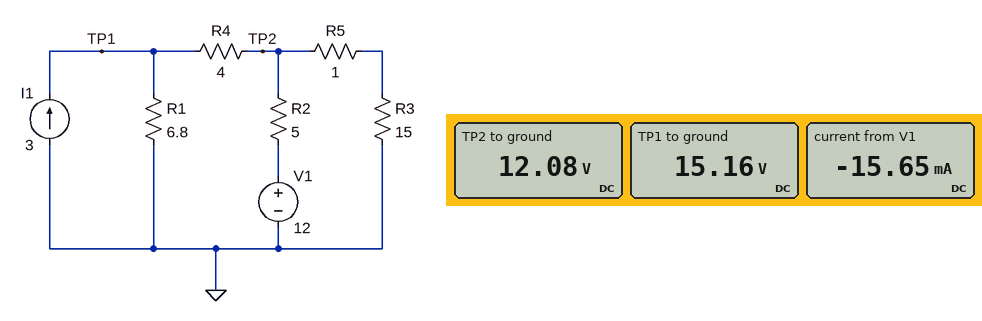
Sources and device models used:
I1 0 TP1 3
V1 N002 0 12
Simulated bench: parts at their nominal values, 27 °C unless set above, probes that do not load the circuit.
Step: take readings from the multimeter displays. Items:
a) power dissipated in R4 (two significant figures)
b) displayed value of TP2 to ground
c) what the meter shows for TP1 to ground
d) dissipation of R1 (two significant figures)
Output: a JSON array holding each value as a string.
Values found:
["2.4 W", "12.08 V", "15.16 V", "34 W"]
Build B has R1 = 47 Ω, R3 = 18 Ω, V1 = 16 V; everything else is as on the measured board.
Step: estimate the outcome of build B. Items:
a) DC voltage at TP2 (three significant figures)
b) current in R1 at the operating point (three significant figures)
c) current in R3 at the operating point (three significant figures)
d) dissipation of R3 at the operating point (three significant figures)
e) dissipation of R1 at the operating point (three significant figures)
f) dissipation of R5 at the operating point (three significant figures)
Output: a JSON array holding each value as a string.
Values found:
["21.9 V", "665 mA", "1.15 A", "23.9 W", "20.8 W", "1.33 W"]
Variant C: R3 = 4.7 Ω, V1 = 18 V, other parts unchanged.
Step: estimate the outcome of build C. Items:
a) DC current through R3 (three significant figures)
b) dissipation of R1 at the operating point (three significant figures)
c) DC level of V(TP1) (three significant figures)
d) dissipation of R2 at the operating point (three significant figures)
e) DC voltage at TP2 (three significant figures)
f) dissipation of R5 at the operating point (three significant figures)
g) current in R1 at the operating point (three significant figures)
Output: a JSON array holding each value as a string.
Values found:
["2.06 A", "32.8 W", "14.9 V", "7.87 W", "11.7 V", "4.23 W", "2.20 A"]
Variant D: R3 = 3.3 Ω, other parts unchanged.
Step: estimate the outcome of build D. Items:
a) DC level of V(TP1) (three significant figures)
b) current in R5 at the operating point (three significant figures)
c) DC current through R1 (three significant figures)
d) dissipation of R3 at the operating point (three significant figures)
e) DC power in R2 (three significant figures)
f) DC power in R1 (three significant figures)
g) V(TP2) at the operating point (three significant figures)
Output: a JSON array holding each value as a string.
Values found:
["12.7 V", "1.90 A", "1.87 A", "11.9 W", "2.94 W", "23.7 W", "8.17 V"]
